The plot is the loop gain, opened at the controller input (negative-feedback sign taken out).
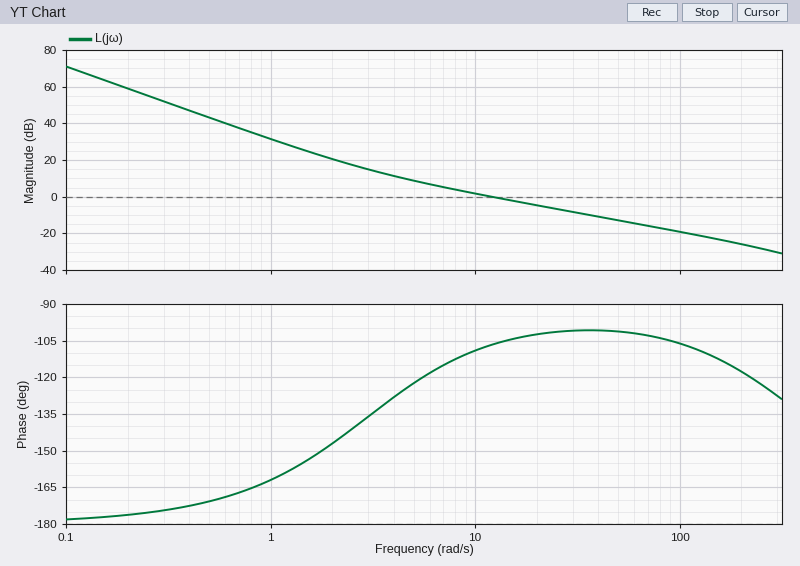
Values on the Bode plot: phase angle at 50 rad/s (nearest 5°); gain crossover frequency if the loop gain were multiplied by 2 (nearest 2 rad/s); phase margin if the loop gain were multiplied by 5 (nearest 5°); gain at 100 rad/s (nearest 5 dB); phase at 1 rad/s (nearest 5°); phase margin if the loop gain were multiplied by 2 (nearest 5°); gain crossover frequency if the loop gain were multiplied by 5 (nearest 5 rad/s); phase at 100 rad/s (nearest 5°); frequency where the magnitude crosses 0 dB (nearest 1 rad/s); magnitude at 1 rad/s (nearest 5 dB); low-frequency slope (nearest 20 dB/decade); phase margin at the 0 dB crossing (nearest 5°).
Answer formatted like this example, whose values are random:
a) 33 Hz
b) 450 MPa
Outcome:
a) -100°
b) 24 rad/s
c) 80°
d) -20 dB
e) -160°
f) 80°
g) 55 rad/s
h) -105°
i) 12 rad/s
j) 30 dB
k) -40 dB/decade
l) 75°
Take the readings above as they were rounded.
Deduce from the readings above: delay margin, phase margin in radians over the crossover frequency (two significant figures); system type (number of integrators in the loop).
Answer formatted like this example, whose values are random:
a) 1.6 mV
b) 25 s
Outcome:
a) 0.11 s
b) 2
